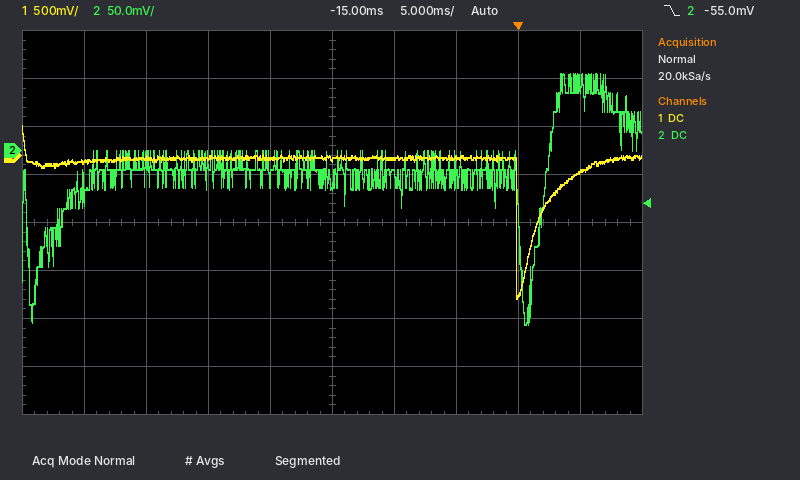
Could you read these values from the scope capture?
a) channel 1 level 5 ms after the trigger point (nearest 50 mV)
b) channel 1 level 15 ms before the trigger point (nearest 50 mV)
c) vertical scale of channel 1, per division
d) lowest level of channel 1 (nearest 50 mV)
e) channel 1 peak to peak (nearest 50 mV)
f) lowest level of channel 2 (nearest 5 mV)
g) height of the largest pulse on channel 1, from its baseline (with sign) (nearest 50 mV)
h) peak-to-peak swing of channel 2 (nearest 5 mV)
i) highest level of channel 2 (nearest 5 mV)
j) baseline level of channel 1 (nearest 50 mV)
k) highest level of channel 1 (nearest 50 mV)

-150 mV
-50 mV
500 mV
-1.50 V
1.80 V
-180 mV
-1.45 V
260 mV
80 mV
-50 mV
300 mV
